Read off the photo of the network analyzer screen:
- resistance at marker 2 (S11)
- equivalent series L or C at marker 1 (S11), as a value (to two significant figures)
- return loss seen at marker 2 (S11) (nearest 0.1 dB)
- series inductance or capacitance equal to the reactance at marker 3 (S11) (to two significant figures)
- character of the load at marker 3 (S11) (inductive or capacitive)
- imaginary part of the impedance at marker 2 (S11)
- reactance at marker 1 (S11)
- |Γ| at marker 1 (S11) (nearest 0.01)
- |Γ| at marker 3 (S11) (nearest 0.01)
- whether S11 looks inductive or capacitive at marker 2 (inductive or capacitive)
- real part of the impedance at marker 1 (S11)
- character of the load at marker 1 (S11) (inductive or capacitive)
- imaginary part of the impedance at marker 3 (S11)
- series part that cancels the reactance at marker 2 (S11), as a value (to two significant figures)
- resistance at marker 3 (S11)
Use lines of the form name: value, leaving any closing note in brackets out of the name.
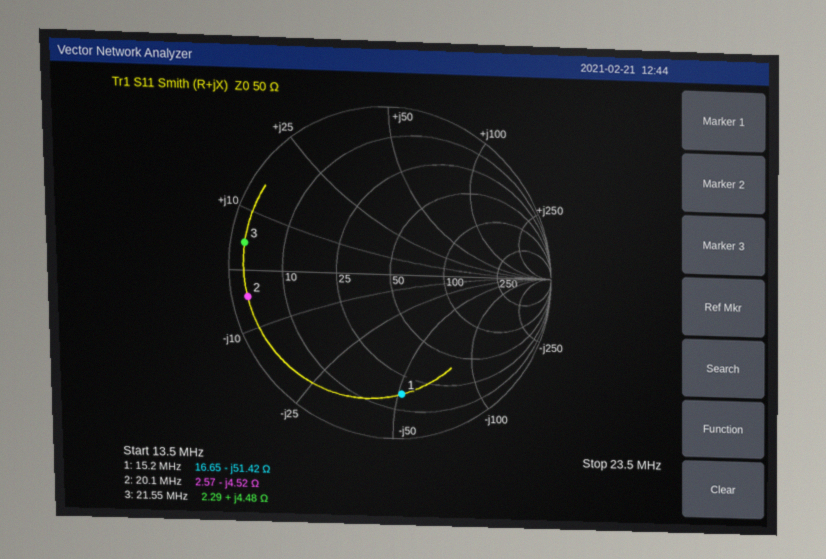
resistance at marker 2: 2.57 Ω
equivalent series L or C at marker 1 (S11), as a value: 200 pF
return loss seen at marker 2 (S11): 0.9 dB
series inductance or capacitance equal to the reactance at marker 3 (S11): 33 nH
character of the load at marker 3 (S11): inductive
imaginary part of the impedance at marker 2: -4.52 Ω
reactance at marker 1: -51.42 Ω
|Γ| at marker 1 (S11): 0.73
|Γ| at marker 3 (S11): 0.91
whether S11 looks inductive or capacitive at marker 2: capacitive
real part of the impedance at marker 1: 16.65 Ω
character of the load at marker 1 (S11): capacitive
imaginary part of the impedance at marker 3: +4.48 Ω
series part that cancels the reactance at marker 2 (S11), as a value: 36 nH
resistance at marker 3: 2.29 Ω
